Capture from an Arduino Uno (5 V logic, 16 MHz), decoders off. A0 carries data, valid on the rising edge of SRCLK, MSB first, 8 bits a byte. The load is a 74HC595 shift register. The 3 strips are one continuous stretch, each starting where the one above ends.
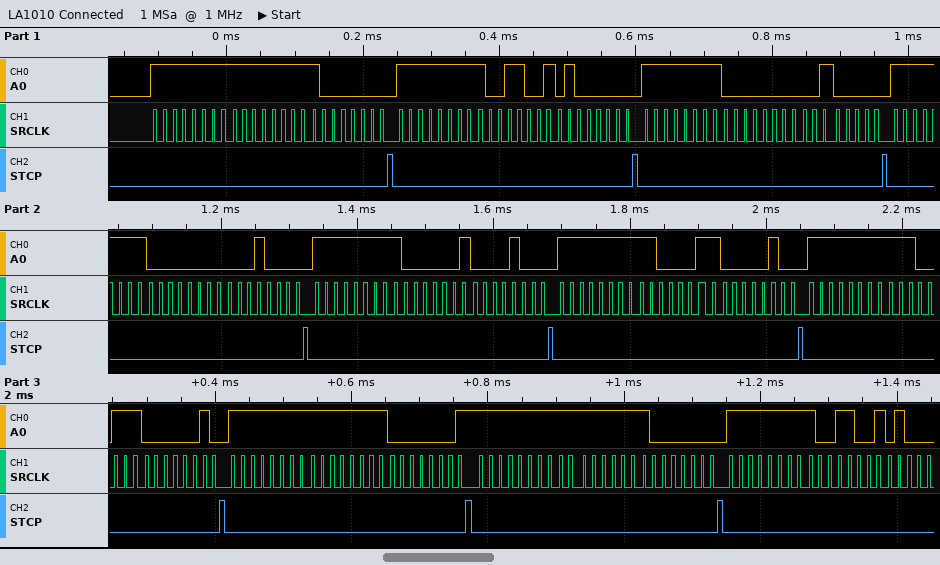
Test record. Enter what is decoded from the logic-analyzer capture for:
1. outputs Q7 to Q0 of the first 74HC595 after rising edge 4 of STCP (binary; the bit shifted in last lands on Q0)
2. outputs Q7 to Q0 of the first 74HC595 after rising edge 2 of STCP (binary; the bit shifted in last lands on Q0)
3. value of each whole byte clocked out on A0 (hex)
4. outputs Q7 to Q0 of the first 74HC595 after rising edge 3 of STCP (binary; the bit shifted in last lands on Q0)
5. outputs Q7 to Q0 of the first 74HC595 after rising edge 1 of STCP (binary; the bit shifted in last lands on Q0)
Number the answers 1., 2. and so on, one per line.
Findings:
1. 00010000
2. 01000000
3. FF FF 80 FF 99 40 FF 00 20 FF 00 10 FF 81 08 FF C3 04 FF E7 02 FF FF 01 FF FF 80 FF 99
4. 00100000
5. 10000000
